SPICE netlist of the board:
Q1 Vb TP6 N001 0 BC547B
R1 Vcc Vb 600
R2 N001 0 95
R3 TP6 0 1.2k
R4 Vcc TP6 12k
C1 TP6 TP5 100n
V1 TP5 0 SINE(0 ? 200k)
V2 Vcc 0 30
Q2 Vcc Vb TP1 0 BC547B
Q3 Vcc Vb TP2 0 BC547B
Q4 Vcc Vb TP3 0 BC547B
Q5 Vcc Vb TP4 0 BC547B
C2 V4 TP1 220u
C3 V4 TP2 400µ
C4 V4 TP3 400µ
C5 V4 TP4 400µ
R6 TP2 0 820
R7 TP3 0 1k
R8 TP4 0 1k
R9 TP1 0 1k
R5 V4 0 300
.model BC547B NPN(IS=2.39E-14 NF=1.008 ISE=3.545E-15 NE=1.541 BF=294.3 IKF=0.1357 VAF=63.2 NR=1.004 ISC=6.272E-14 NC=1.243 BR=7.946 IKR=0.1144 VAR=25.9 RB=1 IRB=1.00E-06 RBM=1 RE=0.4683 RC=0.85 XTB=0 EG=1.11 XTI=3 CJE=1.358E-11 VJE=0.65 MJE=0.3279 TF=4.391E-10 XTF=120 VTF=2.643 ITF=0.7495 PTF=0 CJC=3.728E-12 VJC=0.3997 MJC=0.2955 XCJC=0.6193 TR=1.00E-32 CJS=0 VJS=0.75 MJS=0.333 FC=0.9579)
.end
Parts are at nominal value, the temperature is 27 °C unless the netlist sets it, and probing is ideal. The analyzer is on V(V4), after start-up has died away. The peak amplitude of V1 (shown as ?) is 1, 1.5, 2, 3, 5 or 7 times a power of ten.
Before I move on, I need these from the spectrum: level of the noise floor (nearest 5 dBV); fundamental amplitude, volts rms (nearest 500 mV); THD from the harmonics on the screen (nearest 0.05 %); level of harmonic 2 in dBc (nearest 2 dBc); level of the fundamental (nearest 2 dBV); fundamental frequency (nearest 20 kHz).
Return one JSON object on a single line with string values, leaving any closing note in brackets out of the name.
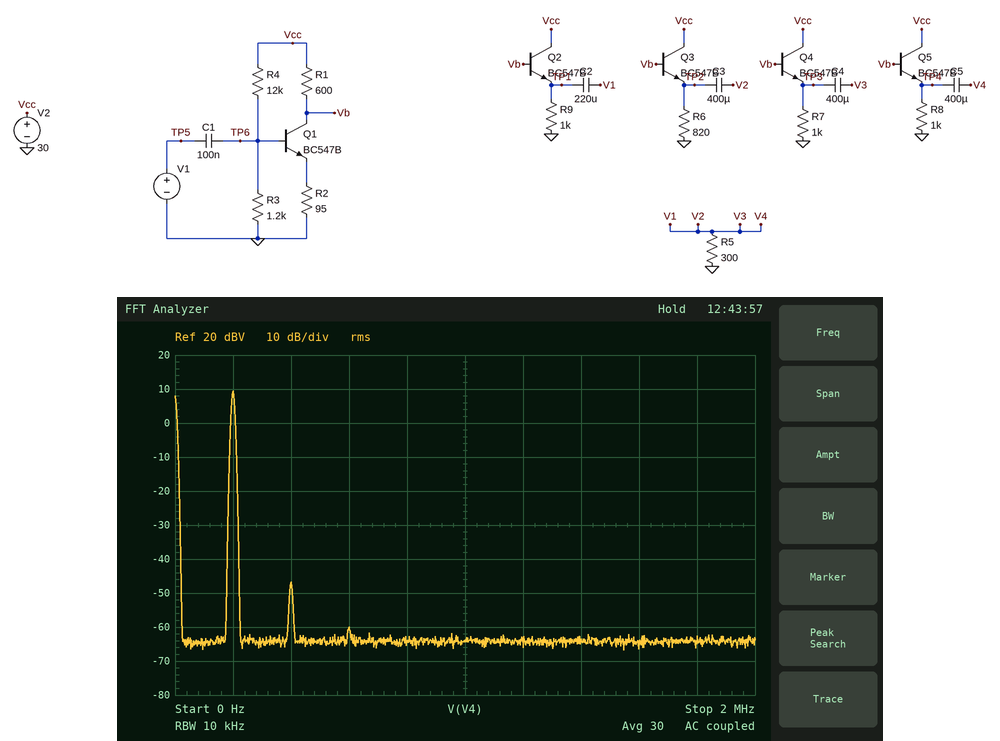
{"level of the noise floor": "-65 dBV", "fundamental amplitude, volts rms": "3.0 V", "THD from the harmonics on the screen": "0.15 %", "level of harmonic 2 in dBc": "-56 dBc", "level of the fundamental": "10 dBV", "fundamental frequency": "200 kHz"}
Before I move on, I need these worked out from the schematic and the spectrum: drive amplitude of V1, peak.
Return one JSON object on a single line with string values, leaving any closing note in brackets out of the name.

{"drive amplitude of V1, peak": "700 mV"}
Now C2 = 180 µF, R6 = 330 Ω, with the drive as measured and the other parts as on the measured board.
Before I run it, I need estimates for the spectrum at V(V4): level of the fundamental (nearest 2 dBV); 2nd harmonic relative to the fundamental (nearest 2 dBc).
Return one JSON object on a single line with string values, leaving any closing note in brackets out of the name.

{"level of the fundamental": "10 dBV", "2nd harmonic relative to the fundamental": "-54 dBc"}
